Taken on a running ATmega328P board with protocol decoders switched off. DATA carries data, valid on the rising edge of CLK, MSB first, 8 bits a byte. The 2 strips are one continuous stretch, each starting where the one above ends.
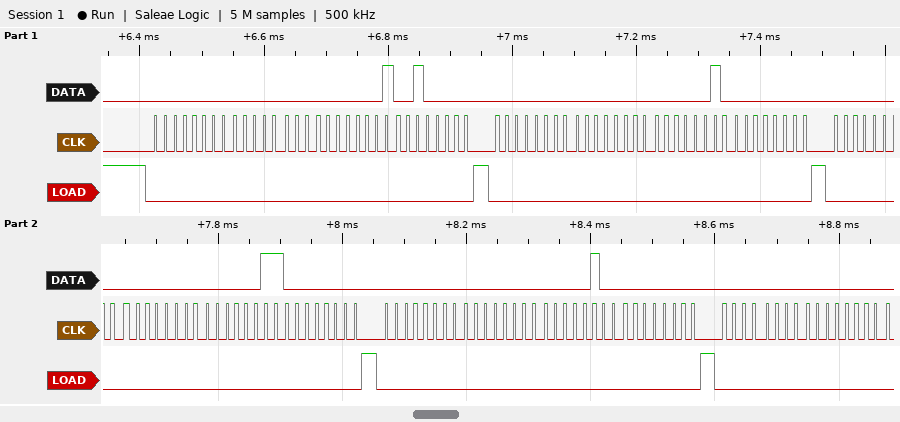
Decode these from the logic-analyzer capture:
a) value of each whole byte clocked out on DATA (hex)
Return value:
00 00 01 20 00 00 02 00 00 00 03 00 00 00 04 00 00 00
